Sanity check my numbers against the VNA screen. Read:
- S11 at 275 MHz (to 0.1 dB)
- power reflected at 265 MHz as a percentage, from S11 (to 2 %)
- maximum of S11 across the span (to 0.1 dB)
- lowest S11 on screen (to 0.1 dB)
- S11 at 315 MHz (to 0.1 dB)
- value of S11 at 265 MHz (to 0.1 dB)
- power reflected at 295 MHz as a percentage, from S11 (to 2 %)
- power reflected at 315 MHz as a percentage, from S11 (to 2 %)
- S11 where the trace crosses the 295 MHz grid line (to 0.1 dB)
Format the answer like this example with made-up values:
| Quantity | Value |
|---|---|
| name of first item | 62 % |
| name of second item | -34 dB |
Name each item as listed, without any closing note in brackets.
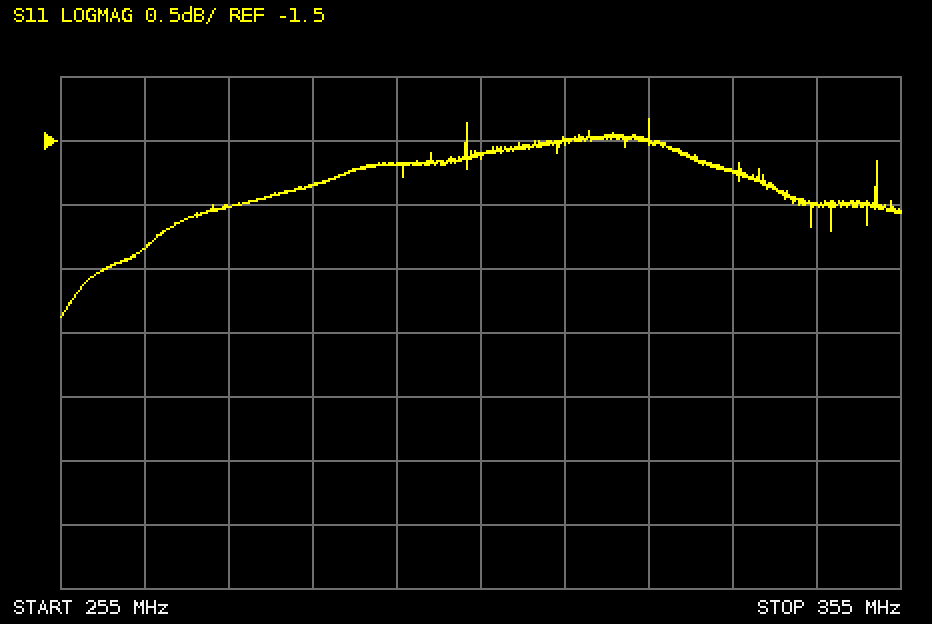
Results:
| Quantity | Value |
|---|---|
| S11 at 275 MHz | -2.0 dB |
| power reflected at 265 MHz as a percentage, from S11 | 58 % |
| maximum of S11 across the span | -1.3 dB |
| lowest S11 on screen | -2.9 dB |
| S11 at 315 MHz | -1.5 dB |
| value of S11 at 265 MHz | -2.3 dB |
| power reflected at 295 MHz as a percentage, from S11 | 68 % |
| power reflected at 315 MHz as a percentage, from S11 | 70 % |
| S11 where the trace crosses the 295 MHz grid line | -1.7 dB |
